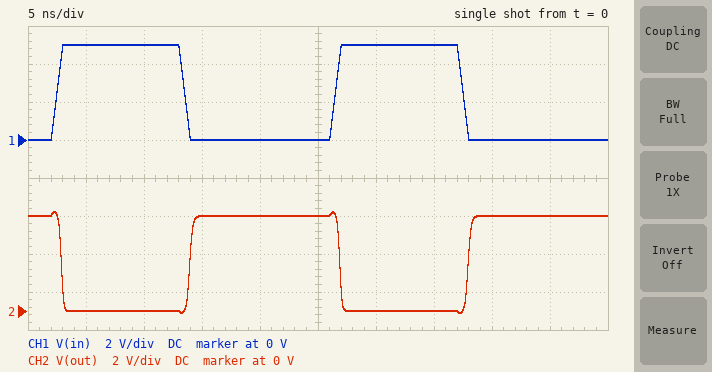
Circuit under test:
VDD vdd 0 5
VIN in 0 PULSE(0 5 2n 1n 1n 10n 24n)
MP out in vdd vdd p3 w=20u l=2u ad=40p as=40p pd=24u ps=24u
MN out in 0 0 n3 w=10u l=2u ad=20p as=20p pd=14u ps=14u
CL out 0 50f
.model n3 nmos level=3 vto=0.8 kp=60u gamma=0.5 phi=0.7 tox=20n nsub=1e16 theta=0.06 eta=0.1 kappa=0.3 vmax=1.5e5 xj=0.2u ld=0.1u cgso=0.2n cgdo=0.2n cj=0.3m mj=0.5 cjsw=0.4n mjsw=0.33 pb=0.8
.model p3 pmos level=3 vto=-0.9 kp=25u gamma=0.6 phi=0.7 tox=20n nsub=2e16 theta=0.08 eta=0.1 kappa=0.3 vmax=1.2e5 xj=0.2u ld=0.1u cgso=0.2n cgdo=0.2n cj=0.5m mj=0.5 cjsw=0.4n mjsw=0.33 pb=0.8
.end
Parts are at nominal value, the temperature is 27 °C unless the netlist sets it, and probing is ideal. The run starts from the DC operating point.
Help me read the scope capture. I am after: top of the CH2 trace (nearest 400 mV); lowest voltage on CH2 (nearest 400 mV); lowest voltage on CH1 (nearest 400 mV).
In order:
5.2 V
0 V
0 V
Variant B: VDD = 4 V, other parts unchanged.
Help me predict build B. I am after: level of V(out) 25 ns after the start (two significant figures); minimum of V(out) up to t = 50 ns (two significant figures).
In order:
4.0 V
-140 mV
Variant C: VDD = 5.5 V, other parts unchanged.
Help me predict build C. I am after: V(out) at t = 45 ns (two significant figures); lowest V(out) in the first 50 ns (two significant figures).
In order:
5.5 V
-81 mV
